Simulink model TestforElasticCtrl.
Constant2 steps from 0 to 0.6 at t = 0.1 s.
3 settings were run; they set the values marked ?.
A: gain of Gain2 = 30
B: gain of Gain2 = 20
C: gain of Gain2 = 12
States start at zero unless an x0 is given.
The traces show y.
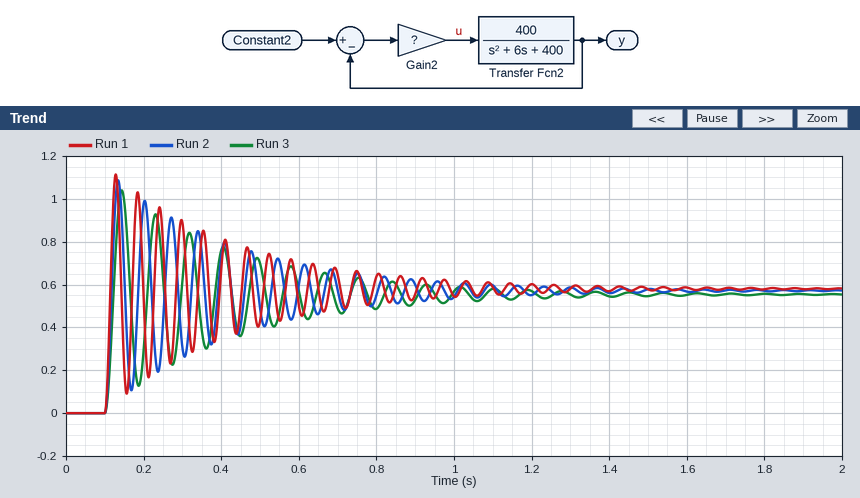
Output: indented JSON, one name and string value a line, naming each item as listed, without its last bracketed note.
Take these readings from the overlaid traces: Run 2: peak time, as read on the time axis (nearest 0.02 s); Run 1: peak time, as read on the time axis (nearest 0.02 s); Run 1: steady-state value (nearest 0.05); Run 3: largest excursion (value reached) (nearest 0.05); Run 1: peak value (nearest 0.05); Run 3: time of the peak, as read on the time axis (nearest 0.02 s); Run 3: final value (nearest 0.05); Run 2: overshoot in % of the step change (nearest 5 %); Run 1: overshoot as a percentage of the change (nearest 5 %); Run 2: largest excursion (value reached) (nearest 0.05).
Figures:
{
  "Run 2: peak time, as read on the time axis": "0.14 s",
  "Run 1: peak time, as read on the time axis": "0.12 s",
  "Run 1: steady-state value": "0.60",
  "Run 3: largest excursion (value reached)": "1.05",
  "Run 1: peak value": "1.10",
  "Run 3: time of the peak, as read on the time axis": "0.14 s",
  "Run 3: final value": "0.55",
  "Run 2: overshoot in % of the step change": "90 %",
  "Run 1: overshoot as a percentage of the change": "90 %",
  "Run 2: largest excursion (value reached)": "1.10"
}
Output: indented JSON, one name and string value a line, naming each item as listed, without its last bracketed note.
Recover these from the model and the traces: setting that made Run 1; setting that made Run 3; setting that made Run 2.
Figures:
{
  "setting that made Run 1": "A",
  "setting that made Run 3": "C",
  "setting that made Run 2": "B"
}
